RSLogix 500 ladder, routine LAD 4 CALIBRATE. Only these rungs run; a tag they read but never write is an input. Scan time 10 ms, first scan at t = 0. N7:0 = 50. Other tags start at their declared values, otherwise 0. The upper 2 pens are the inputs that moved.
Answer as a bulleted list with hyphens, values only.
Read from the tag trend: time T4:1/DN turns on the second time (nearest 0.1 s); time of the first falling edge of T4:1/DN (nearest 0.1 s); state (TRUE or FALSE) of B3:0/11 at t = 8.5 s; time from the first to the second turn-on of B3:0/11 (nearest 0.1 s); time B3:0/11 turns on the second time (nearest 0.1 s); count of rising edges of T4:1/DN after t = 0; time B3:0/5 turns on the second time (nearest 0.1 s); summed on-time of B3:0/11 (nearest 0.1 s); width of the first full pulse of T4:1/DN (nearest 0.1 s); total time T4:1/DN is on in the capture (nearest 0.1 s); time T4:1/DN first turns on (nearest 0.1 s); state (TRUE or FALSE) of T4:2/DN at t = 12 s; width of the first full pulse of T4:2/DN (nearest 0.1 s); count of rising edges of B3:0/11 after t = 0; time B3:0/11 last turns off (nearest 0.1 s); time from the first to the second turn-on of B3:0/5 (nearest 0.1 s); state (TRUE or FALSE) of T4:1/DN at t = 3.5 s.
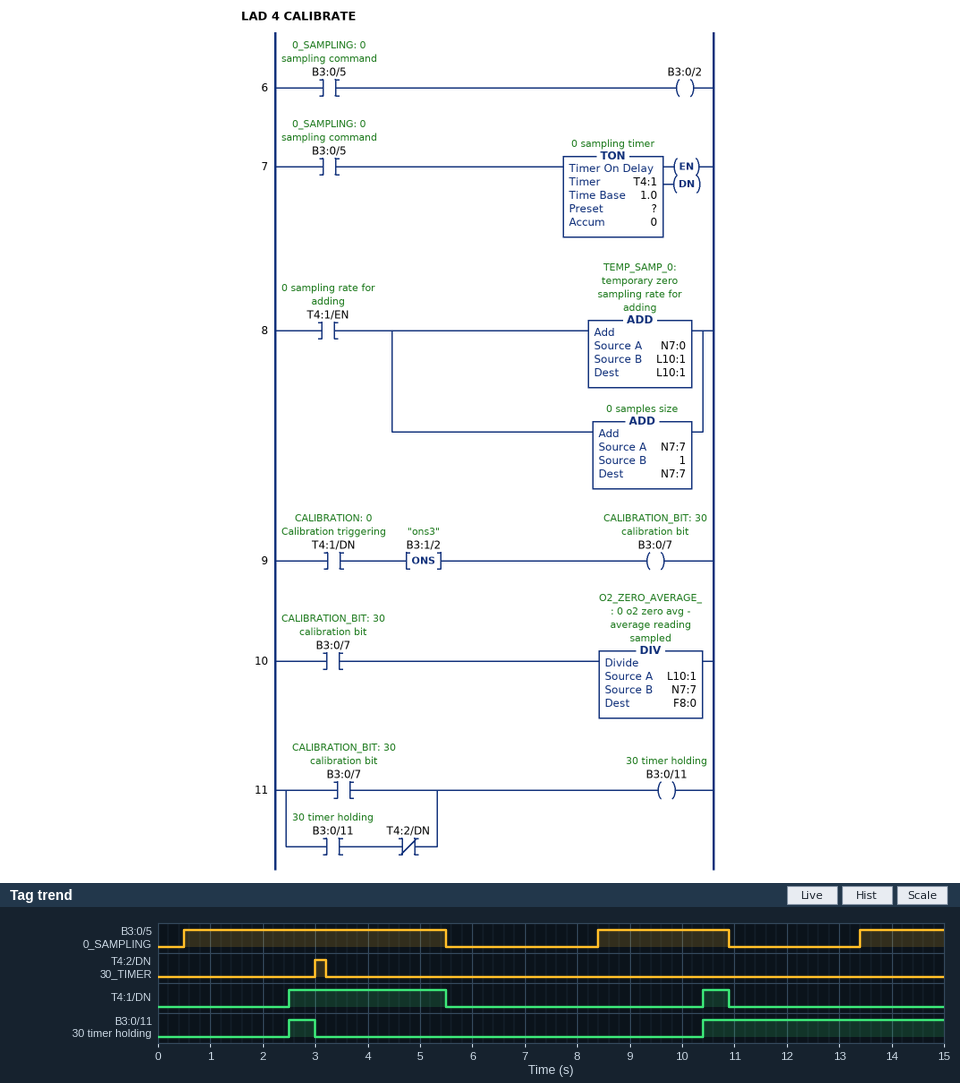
- 10.4 s
- 5.5 s
- FALSE
- 7.9 s
- 10.4 s
- 2
- 8.4 s
- 5.1 s
- 3.0 s
- 3.5 s
- 2.5 s
- FALSE
- 0.2 s
- 2
- 3.0 s
- 7.9 s
- TRUE
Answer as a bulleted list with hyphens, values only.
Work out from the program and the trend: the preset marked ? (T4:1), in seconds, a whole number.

- 2 s
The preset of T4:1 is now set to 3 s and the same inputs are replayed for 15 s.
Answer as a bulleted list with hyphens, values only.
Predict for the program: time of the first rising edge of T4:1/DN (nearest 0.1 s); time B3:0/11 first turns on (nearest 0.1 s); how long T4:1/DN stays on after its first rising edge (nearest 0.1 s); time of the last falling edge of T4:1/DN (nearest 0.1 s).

- 3.5 s
- 3.5 s
- 2.0 s
- 5.5 s
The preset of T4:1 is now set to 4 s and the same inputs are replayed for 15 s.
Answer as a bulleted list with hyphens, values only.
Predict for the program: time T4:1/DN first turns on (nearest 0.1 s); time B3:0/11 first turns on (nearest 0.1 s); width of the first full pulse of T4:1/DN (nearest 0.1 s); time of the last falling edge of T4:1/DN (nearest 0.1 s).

- 4.5 s
- 4.5 s
- 1.0 s
- 5.5 s
